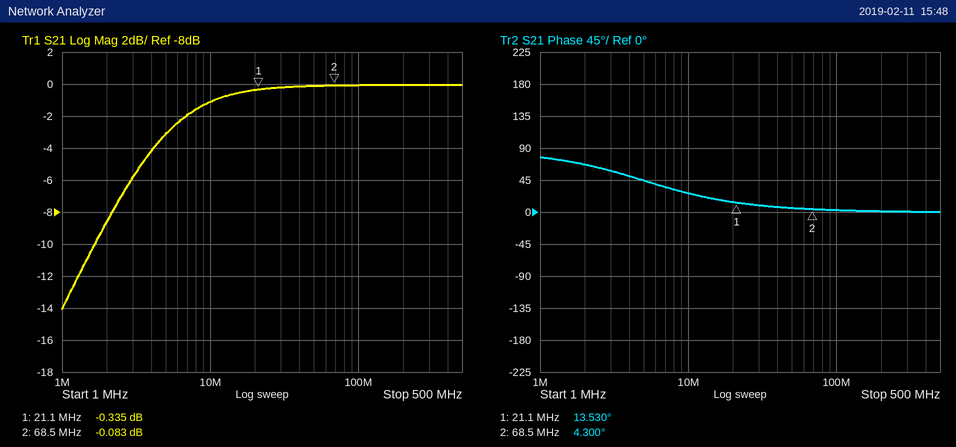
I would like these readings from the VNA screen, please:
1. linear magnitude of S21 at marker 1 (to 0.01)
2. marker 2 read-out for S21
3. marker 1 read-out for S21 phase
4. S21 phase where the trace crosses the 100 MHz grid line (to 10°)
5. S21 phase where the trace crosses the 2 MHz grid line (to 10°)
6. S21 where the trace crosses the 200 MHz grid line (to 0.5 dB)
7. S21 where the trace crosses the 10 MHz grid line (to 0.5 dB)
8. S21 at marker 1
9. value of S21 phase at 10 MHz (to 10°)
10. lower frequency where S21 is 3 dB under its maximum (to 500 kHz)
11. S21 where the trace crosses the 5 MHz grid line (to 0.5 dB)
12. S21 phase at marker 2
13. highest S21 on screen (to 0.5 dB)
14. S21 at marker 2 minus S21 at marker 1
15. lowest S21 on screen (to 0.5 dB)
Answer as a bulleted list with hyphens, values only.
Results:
- 0.96
- -0.083 dB
- 13.530°
- 0°
- 70°
- 0.0 dB
- -1.0 dB
- -0.335 dB
- 30°
- 5.0 MHz
- -3.0 dB
- 4.300°
- 0.0 dB
- 0.252 dB
- -14.0 dB
